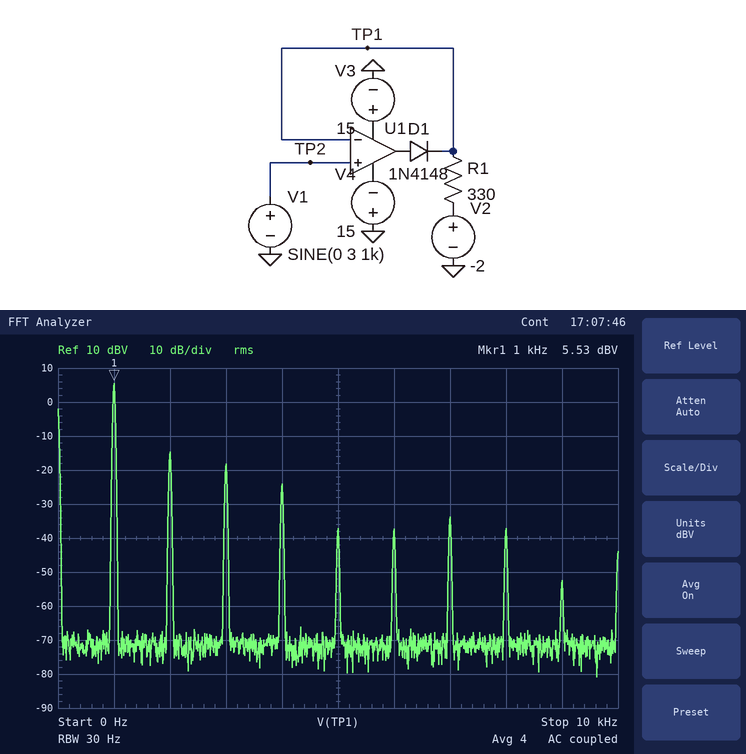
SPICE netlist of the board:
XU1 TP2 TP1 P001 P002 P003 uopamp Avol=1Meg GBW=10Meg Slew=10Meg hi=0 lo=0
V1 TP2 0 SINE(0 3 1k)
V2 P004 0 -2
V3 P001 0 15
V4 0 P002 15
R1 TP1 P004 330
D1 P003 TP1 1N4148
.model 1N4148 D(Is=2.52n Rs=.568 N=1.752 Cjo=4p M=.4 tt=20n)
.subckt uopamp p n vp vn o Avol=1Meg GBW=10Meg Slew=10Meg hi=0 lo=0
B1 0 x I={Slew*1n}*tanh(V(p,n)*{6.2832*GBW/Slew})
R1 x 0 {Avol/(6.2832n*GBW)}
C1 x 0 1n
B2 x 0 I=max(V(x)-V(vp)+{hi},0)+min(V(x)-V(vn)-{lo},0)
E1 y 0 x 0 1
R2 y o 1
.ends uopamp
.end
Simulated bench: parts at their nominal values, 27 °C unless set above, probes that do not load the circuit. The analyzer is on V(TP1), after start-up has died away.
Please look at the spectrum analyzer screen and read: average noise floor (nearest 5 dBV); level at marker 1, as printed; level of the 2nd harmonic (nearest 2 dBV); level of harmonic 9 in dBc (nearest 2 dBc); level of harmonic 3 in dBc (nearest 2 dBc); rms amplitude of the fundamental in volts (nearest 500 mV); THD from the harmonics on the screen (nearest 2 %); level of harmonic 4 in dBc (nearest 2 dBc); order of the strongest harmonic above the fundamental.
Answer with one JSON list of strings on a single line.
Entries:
["-70 dBV", "5.53 dBV", "-14 dBV", "-58 dBc", "-24 dBc", "2.0 V", "12 %", "-30 dBc", "2"]
